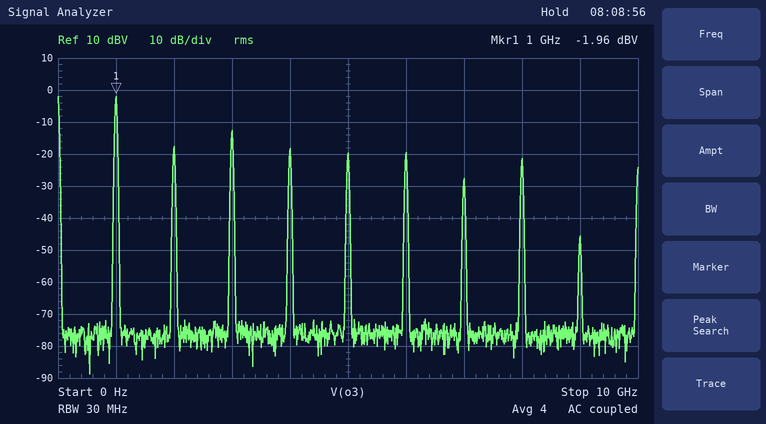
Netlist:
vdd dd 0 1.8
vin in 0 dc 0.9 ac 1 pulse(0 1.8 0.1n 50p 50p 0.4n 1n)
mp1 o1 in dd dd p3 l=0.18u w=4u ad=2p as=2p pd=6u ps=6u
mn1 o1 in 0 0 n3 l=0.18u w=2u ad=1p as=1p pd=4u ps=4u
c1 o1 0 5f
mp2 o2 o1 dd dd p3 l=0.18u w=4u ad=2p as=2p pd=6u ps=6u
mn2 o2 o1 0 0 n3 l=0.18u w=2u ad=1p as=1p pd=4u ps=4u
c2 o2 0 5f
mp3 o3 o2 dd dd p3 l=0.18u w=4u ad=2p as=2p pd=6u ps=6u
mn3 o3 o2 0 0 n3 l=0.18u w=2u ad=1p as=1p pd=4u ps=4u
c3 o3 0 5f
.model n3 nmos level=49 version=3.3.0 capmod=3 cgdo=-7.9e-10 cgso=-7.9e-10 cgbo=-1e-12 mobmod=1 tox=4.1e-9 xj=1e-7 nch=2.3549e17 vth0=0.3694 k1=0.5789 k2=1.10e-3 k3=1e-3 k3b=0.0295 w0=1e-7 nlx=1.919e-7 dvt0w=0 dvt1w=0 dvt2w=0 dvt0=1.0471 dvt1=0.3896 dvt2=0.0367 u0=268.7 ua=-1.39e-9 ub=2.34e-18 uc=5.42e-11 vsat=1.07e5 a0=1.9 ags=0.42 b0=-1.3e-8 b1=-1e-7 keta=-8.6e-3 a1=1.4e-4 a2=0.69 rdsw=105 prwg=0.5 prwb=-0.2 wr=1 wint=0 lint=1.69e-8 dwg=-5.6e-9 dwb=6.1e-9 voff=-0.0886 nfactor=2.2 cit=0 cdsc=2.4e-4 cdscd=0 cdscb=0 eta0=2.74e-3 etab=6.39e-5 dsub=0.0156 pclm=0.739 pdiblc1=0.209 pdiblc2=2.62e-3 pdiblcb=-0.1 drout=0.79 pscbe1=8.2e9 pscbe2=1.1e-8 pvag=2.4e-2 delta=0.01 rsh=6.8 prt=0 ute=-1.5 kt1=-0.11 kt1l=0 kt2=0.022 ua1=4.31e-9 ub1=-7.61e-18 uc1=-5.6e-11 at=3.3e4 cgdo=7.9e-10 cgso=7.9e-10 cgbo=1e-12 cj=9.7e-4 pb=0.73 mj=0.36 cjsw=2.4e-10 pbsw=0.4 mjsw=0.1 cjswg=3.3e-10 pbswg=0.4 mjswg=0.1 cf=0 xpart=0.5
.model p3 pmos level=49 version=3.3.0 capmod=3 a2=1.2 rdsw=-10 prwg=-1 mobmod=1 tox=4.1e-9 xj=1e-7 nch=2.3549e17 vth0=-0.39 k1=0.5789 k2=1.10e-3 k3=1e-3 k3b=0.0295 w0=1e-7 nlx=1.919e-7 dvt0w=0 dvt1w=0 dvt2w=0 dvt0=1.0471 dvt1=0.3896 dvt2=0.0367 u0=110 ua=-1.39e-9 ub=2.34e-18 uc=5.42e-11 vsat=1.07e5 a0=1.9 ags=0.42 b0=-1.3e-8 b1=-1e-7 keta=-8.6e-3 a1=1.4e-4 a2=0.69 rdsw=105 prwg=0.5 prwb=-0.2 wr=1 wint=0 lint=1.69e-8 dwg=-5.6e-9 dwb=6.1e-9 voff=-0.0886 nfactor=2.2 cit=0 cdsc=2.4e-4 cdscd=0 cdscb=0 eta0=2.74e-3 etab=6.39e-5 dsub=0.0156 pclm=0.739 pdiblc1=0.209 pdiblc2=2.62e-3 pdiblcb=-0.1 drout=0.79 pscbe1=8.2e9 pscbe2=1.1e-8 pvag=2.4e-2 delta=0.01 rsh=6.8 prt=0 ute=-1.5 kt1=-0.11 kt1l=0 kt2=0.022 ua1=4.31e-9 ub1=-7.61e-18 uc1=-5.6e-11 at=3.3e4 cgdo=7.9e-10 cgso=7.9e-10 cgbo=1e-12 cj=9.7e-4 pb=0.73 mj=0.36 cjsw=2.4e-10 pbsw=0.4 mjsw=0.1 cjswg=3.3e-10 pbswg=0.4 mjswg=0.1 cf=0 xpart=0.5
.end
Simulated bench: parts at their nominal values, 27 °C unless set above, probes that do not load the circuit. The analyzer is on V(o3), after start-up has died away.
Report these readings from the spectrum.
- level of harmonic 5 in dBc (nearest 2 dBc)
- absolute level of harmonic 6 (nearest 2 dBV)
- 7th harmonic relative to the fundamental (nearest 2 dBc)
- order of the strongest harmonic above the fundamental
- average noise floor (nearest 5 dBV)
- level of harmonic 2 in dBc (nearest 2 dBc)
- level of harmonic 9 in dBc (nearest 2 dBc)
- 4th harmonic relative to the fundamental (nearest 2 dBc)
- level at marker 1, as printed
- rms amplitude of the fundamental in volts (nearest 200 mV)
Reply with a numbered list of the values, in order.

1. -18 dBc
2. -20 dBV
3. -26 dBc
4. 3
5. -75 dBV
6. -16 dBc
7. -44 dBc
8. -16 dBc
9. -1.96 dBV
10. 800 mV
